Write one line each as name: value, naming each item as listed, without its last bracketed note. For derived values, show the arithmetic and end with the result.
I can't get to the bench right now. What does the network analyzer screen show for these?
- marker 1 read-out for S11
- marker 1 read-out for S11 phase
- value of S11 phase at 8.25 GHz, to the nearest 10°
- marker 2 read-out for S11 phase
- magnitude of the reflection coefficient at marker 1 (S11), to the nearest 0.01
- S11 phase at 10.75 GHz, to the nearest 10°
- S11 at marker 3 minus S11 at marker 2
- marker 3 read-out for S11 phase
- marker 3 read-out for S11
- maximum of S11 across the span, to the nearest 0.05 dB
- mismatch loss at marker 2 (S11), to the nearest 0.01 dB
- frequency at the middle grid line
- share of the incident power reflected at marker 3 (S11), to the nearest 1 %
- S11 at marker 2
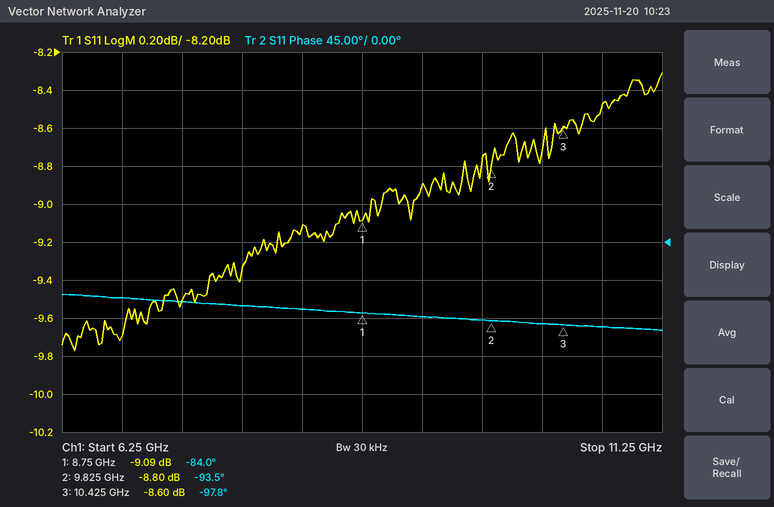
marker 1 read-out for S11: -9.09 dB
marker 1 read-out for S11 phase: -84.0°
value of S11 phase at 8.25 GHz, to the nearest 10°: -80°
marker 2 read-out for S11 phase: -93.5°
magnitude of the reflection coefficient at marker 1 (S11), to the nearest 0.01: 10^(-9.09/20) ≈ 0.35
S11 phase at 10.75 GHz, to the nearest 10°: -100°
S11 at marker 3 minus S11 at marker 2: -8.6 − (-8.8) = 0.20 dB
marker 3 read-out for S11 phase: -97.8°
marker 3 read-out for S11: -8.60 dB
maximum of S11 across the span, to the nearest 0.05 dB: -8.30 dB
mismatch loss at marker 2 (S11), to the nearest 0.01 dB: −10 log10(1 − 10^(-8.8/10)) ≈ 0.61 dB
frequency at the middle grid line: 8.75 GHz
share of the incident power reflected at marker 3 (S11), to the nearest 1 %: 10^(-8.6/10) ≈ 14 %
S11 at marker 2: -8.80 dB
